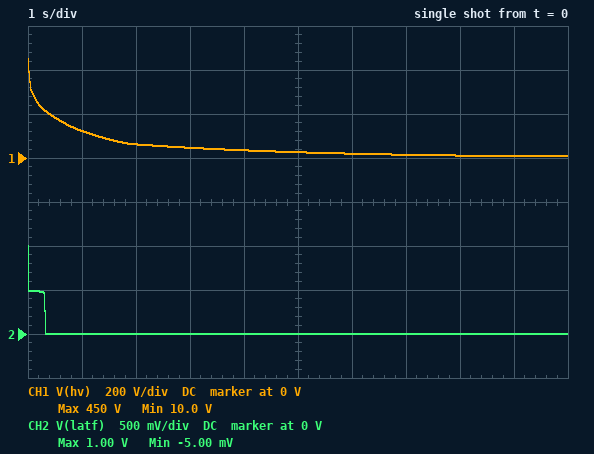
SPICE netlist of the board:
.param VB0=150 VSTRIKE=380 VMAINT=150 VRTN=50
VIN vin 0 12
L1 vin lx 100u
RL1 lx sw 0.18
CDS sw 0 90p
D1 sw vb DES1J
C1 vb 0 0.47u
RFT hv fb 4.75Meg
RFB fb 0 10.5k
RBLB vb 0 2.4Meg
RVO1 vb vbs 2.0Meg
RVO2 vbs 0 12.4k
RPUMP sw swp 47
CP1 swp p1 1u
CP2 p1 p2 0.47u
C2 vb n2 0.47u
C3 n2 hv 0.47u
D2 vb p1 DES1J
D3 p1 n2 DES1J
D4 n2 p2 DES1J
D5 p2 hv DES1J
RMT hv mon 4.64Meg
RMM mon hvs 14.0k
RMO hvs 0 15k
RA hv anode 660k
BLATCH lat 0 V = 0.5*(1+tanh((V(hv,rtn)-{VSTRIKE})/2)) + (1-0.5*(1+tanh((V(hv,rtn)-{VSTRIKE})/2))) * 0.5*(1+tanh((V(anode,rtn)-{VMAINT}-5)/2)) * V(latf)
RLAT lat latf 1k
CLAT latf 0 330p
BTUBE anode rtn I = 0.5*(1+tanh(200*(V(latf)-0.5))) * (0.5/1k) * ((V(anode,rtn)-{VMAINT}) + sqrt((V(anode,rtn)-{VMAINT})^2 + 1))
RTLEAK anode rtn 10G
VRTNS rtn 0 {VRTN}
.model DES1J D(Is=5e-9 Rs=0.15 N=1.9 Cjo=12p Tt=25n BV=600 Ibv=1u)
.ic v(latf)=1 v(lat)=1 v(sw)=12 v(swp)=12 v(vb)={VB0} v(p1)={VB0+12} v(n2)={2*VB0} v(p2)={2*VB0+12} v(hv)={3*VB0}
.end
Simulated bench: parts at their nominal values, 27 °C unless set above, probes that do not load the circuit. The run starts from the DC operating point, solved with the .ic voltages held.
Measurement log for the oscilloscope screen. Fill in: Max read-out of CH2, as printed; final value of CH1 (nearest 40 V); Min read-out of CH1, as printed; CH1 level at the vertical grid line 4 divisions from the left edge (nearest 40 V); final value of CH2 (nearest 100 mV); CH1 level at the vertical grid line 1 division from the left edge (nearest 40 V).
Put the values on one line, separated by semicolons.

1.00 V; 0 V; 10.0 V; 40 V; 0 V; 120 V
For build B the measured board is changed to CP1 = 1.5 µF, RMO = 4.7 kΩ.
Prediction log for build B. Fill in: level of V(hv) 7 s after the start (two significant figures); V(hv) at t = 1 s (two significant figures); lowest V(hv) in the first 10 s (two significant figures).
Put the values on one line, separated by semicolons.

28 V; 130 V; 15 V
